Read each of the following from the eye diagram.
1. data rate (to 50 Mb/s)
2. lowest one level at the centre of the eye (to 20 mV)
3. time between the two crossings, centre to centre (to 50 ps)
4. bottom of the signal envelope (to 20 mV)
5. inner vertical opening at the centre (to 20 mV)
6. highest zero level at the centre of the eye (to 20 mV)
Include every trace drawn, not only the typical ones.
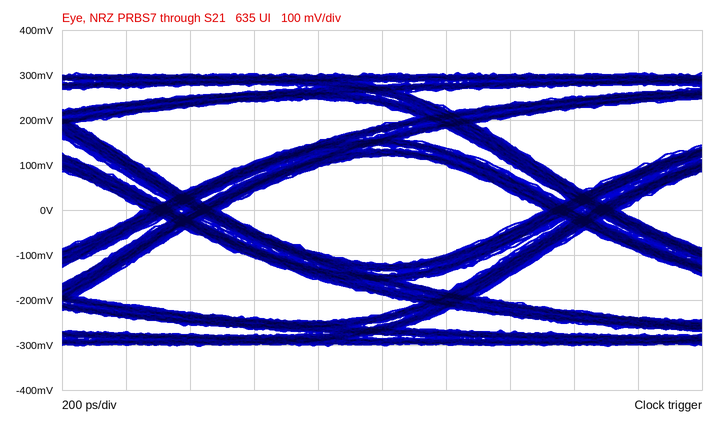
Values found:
800 Mb/s
120 mV
1.25 ns
-300 mV
240 mV
-120 mV
